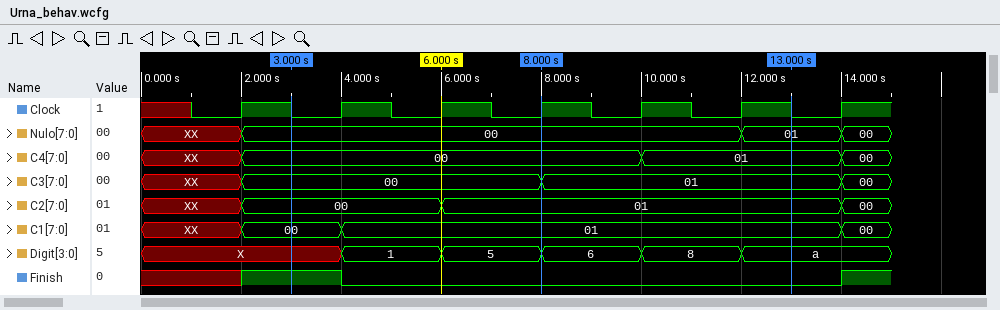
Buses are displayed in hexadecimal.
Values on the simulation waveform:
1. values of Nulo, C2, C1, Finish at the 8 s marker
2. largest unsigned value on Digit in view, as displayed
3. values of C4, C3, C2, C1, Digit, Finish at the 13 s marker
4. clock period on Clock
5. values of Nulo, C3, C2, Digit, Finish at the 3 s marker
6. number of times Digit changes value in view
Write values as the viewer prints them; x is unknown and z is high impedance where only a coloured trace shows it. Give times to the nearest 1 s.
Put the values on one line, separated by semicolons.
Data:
Nulo=00, C2=01, C1=01, Finish=0; a; C4=01, C3=01, C2=01, C1=01, Digit=a, Finish=0; 2 s; Nulo=00, C3=00, C2=00, Digit=X, Finish=1; 5
